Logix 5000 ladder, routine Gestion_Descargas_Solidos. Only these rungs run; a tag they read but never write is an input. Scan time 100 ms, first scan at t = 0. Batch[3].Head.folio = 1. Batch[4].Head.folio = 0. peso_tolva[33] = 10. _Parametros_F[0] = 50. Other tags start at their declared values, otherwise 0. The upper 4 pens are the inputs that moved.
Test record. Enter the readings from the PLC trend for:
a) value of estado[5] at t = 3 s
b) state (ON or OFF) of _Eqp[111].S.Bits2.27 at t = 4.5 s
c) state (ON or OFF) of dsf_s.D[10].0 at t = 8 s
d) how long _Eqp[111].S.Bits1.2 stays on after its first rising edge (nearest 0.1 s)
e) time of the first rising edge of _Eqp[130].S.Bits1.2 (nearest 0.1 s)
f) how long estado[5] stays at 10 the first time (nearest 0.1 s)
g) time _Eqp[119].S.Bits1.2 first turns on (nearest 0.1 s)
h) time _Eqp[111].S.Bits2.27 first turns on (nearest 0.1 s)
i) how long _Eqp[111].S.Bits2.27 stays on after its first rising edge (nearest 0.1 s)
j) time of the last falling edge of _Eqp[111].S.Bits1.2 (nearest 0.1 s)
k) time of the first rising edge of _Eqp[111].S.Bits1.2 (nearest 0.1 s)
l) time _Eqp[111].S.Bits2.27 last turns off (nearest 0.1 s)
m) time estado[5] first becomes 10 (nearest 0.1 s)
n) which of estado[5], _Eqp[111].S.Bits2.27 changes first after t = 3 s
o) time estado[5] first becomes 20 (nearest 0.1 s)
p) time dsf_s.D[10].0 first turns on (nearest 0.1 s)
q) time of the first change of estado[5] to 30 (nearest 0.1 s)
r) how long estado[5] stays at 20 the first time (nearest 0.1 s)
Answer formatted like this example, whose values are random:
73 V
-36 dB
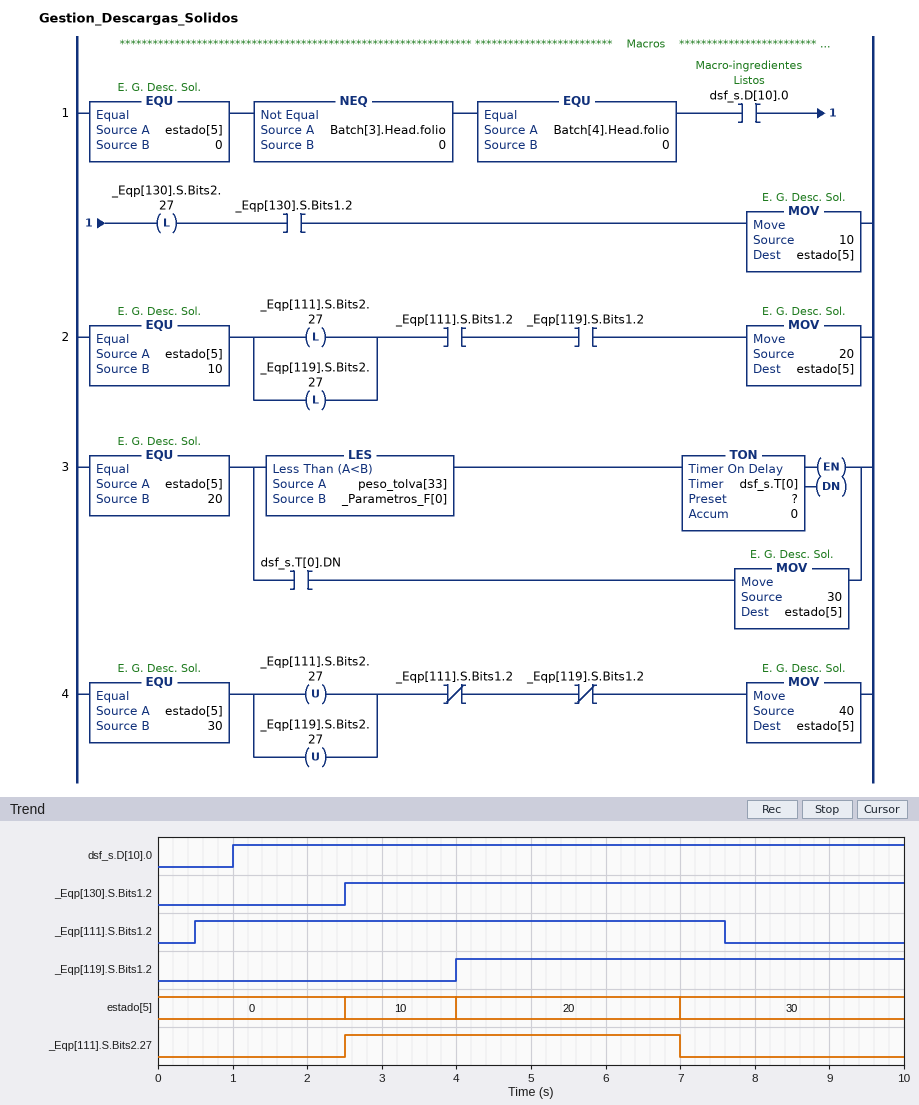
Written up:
10
ON
ON
7.1 s
2.5 s
1.5 s
4.0 s
2.5 s
4.5 s
7.6 s
0.5 s
7.0 s
2.5 s
estado[5]
4.0 s
1.0 s
7.0 s
3.0 s
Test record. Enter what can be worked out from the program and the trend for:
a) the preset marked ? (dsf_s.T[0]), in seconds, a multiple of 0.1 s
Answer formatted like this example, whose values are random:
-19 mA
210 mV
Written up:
3.0 s
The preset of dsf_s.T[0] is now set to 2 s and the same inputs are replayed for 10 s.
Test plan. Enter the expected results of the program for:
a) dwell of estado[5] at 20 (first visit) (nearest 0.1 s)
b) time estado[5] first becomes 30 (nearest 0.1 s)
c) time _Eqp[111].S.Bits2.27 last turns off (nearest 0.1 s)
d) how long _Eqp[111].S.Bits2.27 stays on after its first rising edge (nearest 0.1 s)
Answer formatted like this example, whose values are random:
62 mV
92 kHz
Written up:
2.0 s
6.0 s
6.0 s
3.5 s
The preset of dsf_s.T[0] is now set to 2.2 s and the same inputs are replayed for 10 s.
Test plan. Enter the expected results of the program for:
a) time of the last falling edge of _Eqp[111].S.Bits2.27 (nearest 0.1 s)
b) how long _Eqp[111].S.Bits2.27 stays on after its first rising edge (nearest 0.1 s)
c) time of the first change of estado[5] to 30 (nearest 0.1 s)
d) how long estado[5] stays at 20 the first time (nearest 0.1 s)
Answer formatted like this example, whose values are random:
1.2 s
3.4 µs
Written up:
6.2 s
3.7 s
6.2 s
2.2 s
